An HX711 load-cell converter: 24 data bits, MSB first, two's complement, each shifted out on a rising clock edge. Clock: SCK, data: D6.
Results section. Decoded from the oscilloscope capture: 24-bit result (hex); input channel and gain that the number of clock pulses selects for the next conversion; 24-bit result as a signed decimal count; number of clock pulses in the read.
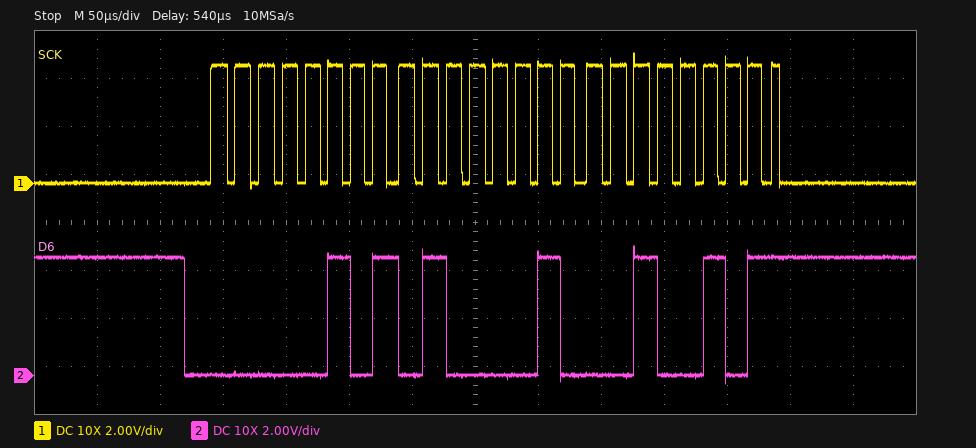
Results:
0x054225
channel A, gain 128
344613
25
